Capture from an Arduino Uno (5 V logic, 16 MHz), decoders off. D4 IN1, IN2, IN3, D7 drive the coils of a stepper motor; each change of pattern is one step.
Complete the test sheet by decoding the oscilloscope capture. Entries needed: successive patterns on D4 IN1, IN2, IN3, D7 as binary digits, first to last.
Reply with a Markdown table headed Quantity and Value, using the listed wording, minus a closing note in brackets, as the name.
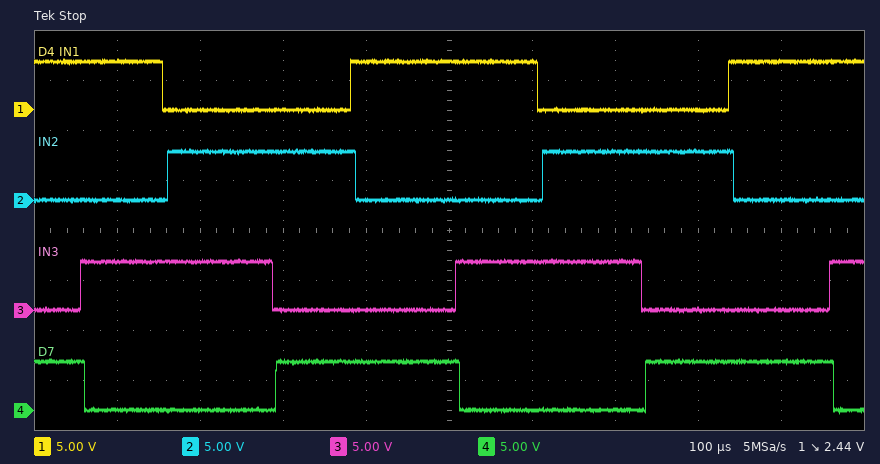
| Quantity | Value |
|---|---|
| successive patterns on D4 IN1, IN2, IN3, D7 as binary digits, first to last | 1001 1010 0110 0101 1001 1010 0110 0101 1001 1010 |
